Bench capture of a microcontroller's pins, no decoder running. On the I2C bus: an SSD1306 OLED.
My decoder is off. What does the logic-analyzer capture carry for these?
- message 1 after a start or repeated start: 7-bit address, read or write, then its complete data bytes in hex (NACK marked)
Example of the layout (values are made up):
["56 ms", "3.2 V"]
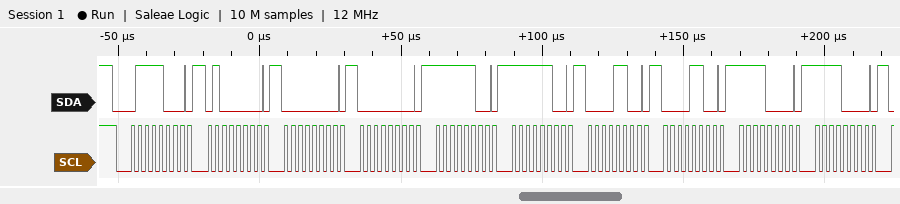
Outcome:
["0x3C write: 40 00 00 FC FC 0C 0C F0 F0"]
